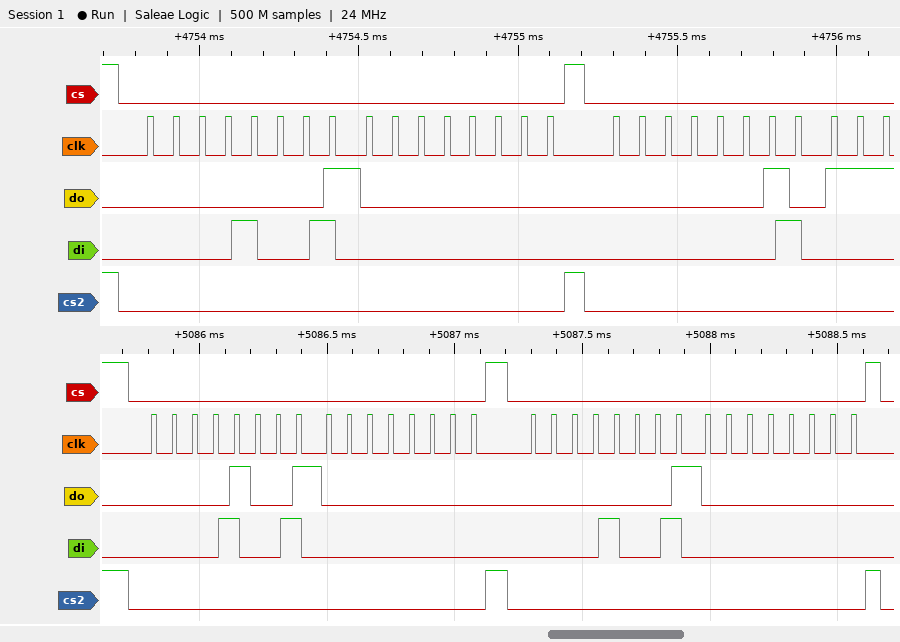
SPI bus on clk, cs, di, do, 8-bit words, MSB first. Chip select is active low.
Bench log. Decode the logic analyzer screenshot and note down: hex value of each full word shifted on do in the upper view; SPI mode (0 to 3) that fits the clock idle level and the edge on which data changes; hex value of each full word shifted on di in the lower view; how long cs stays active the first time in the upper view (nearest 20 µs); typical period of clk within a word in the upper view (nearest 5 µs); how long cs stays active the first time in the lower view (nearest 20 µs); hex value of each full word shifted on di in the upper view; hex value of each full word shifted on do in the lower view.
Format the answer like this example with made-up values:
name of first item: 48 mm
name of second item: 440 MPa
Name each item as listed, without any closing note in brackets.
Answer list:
hex value of each full word shifted on do in the upper view: 01, 00, 02
SPI mode (0 to 3) that fits the clock idle level and the edge on which data changes: 0
hex value of each full word shifted on di in the lower view: 09, 00, 09, 00
how long cs stays active the first time in the upper view: 1400 µs
typical period of clk within a word in the upper view: 80 µs
how long cs stays active the first time in the lower view: 1400 µs
hex value of each full word shifted on di in the upper view: 09, 00, 01
hex value of each full word shifted on do in the lower view: 09, 00, 01, 00
